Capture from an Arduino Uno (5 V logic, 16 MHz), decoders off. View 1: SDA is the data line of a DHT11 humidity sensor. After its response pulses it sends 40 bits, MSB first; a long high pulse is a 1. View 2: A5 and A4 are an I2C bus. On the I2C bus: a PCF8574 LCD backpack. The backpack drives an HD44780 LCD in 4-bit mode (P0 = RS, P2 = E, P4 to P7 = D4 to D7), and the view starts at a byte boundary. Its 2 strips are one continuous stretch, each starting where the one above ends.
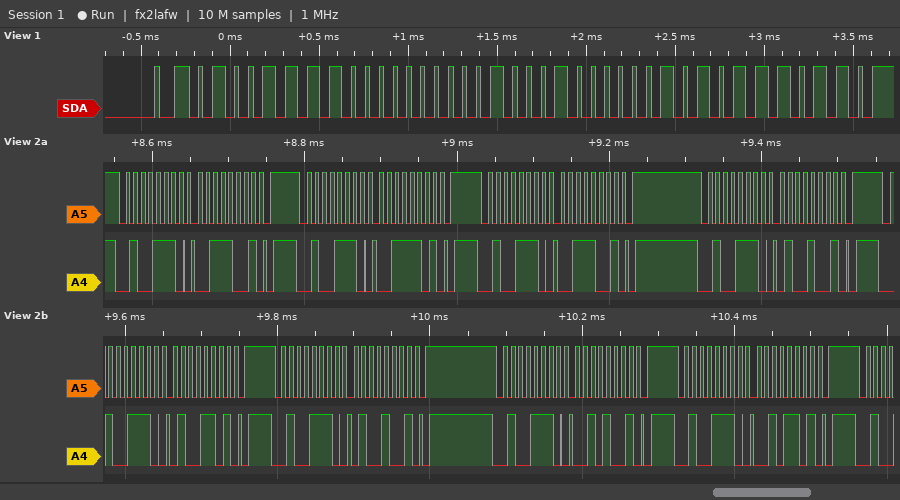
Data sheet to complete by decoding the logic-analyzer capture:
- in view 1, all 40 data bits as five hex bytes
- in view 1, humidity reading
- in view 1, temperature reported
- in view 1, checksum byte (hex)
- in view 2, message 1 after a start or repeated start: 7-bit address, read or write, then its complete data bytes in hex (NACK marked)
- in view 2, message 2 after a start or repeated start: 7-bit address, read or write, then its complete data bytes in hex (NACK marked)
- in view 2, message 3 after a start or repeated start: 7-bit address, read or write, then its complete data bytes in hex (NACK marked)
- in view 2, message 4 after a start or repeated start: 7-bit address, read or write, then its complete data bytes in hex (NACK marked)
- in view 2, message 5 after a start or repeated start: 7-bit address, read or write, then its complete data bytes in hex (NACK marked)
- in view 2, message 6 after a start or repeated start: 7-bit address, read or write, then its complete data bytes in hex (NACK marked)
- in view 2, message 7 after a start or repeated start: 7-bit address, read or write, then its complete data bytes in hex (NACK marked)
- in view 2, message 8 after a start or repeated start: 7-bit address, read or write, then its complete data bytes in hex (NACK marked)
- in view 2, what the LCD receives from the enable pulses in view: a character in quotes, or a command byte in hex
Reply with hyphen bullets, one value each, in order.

- 4F 00 22 05 76
- 79 %
- 34.5 °C
- 0x76
- 0x27 write: 39
- 0x27 write: 3D
- 0x27 write: 39
- 0x27 write: 49
- 0x27 write: 4D
- 0x27 write: 49
- 0x27 write: 29
- 0x27 write: 2D
- '4'
